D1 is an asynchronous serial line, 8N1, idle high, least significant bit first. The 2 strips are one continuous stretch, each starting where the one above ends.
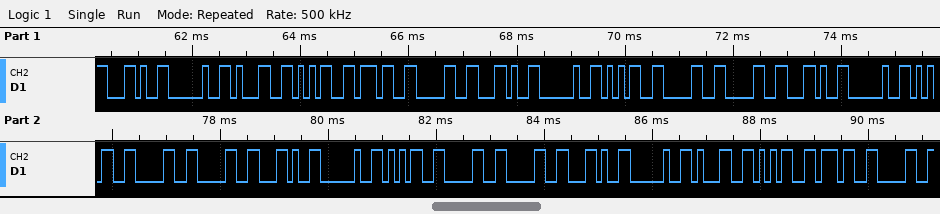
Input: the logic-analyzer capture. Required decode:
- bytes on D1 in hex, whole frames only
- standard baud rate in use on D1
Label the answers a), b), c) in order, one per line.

a) 2C 20 31 35 37 30 2C 20 35 30 30 2C 20 35 30 30 2C 20 35 30 30 2C 20 31 35 37 30
b) 9600 baud
